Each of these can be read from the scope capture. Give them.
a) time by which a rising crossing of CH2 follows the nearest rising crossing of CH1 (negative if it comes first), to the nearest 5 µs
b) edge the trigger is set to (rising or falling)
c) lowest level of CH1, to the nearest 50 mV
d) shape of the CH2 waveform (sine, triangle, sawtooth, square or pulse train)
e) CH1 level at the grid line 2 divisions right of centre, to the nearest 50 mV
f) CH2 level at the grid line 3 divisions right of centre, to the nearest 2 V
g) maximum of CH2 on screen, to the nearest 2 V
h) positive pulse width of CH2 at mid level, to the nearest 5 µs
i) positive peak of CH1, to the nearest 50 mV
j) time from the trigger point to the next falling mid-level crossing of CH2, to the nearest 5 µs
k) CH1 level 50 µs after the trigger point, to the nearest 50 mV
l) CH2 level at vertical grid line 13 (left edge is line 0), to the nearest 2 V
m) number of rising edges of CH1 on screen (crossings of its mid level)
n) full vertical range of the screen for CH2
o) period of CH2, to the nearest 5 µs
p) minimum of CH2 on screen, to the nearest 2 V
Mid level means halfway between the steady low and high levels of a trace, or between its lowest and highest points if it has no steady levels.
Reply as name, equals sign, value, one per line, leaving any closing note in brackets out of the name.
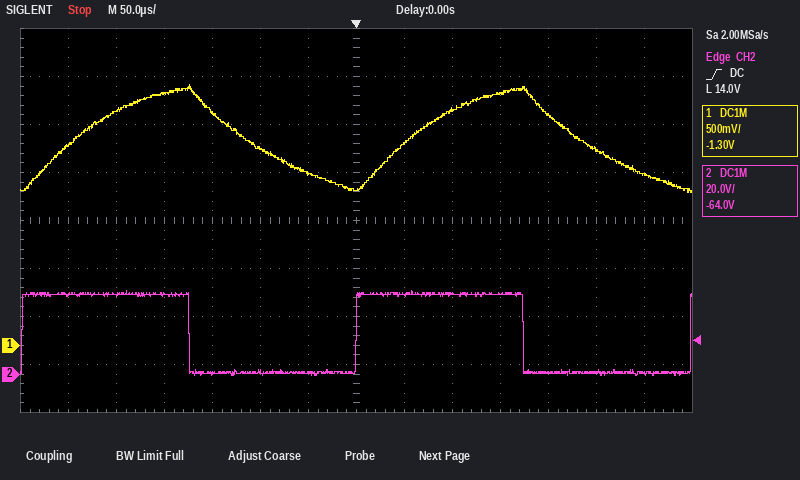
time by which a rising crossing of CH2 follows the nearest rising crossing of CH1 (negative if it comes first), to the nearest 5 µs = -55 µs
edge the trigger is set to = rising
lowest level of CH1, to the nearest 50 mV = 1.60 V
shape of the CH2 waveform = square
CH1 level at the grid line 2 divisions right of centre, to the nearest 50 mV = 2.45 V
CH2 level at the grid line 3 divisions right of centre, to the nearest 2 V = 34 V
maximum of CH2 on screen, to the nearest 2 V = 34 V
positive pulse width of CH2 at mid level, to the nearest 5 µs = 175 µs
positive peak of CH1, to the nearest 50 mV = 2.70 V
time from the trigger point to the next falling mid-level crossing of CH2, to the nearest 5 µs = 175 µs
CH1 level 50 µs after the trigger point, to the nearest 50 mV = 2.10 V
CH2 level at vertical grid line 13 (left edge is line 0), to the nearest 2 V = 0 V
number of rising edges of CH1 on screen = 2
full vertical range of the screen for CH2 = 160 V
period of CH2, to the nearest 5 µs = 350 µs
minimum of CH2 on screen, to the nearest 2 V = 0 V
